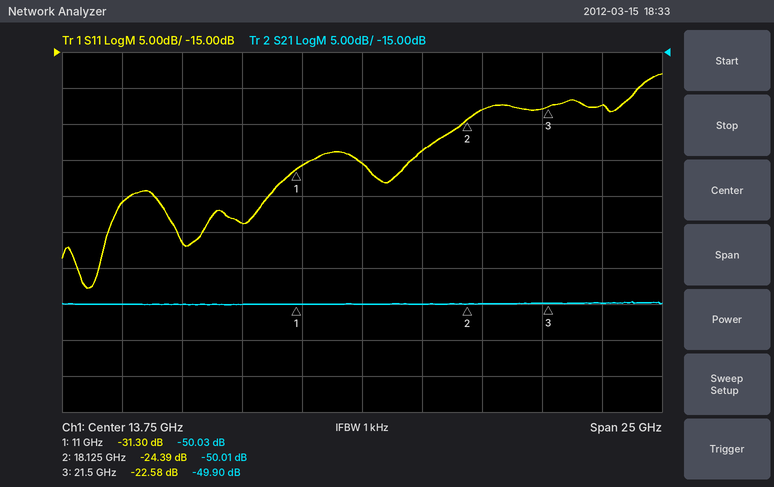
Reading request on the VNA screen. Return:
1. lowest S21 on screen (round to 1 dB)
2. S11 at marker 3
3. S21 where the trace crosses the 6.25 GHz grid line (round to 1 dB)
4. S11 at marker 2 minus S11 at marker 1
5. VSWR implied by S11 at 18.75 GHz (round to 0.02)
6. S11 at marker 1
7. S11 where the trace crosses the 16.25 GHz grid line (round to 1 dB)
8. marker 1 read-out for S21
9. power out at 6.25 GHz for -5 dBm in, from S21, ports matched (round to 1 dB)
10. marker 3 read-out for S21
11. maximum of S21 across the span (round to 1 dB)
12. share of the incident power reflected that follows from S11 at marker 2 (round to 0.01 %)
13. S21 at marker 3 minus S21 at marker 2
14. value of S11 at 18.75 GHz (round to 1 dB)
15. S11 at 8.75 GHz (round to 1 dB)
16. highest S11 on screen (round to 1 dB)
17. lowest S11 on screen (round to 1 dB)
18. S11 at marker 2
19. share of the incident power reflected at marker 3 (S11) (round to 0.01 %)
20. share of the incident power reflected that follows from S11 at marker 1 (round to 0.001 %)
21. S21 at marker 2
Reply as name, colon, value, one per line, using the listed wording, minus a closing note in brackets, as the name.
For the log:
lowest S21 on screen: -50 dB
S11 at marker 3: -22.58 dB
S21 where the trace crosses the 6.25 GHz grid line: -50 dB
S11 at marker 2 minus S11 at marker 1: 6.91 dB
VSWR implied by S11 at 18.75 GHz: 1.16
S11 at marker 1: -31.30 dB
S11 where the trace crosses the 16.25 GHz grid line: -29 dB
marker 1 read-out for S21: -50.03 dB
power out at 6.25 GHz for -5 dBm in, from S21, ports matched: -55 dBm
marker 3 read-out for S21: -49.90 dB
maximum of S21 across the span: -50 dB
share of the incident power reflected that follows from S11 at marker 2: 0.36 %
S21 at marker 3 minus S21 at marker 2: 0.11 dB
value of S11 at 18.75 GHz: -23 dB
S11 at 8.75 GHz: -39 dB
highest S11 on screen: -18 dB
lowest S11 on screen: -48 dB
S11 at marker 2: -24.39 dB
share of the incident power reflected at marker 3 (S11): 0.55 %
share of the incident power reflected that follows from S11 at marker 1: 0.074 %
S21 at marker 2: -50.01 dB
